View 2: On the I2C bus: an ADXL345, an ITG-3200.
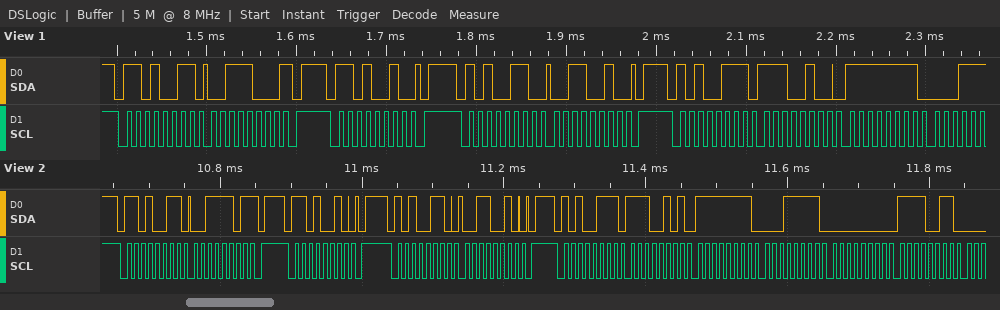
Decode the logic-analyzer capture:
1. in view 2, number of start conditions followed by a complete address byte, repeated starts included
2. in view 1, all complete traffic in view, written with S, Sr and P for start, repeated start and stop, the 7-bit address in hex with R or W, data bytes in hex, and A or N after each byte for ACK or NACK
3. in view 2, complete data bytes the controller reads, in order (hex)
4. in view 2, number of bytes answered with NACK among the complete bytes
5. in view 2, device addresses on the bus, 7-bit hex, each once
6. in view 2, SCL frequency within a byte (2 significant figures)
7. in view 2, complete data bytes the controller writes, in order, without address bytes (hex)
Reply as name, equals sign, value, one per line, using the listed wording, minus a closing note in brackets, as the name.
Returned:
in view 2, number of start conditions followed by a complete address byte, repeated starts included = 4
in view 1, all complete traffic in view, written with S, Sr and P for start, repeated start and stop, the 7-bit address in hex with R or W, data bytes in hex, and A or N after each byte for ACK or NACK = S 69R A 38 N P S 69W A P S 53W A 32 A P S 53R A E4 A FF A
in view 2, complete data bytes the controller reads, in order = 3D E5 FF 1F 00 F3
in view 2, number of bytes answered with NACK among the complete bytes = 1
in view 2, device addresses on the bus, 7-bit hex, each once = 0x69 0x53
in view 2, SCL frequency within a byte = 100 kHz
in view 2, complete data bytes the controller writes, in order, without address bytes = 32
